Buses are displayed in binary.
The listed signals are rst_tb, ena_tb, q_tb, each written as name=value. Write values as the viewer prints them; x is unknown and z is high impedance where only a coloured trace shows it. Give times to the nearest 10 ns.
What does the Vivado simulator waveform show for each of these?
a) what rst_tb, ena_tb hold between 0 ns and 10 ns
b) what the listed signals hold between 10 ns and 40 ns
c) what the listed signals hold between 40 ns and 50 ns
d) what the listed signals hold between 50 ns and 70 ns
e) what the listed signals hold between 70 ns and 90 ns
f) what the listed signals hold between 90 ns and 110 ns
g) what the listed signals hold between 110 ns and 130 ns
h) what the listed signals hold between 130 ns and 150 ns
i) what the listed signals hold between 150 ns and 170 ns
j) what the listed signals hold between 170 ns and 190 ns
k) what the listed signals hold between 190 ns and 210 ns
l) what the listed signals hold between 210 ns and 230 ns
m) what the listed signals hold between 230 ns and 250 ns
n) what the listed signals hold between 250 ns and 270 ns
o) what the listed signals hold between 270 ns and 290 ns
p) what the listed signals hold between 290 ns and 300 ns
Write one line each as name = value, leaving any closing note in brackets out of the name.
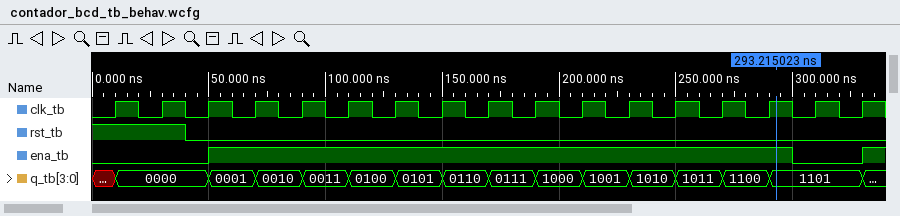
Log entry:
what rst_tb, ena_tb hold between 0 ns and 10 ns = rst_tb=1, ena_tb=0
what the listed signals hold between 10 ns and 40 ns = rst_tb=1, ena_tb=0, q_tb=0000
what the listed signals hold between 40 ns and 50 ns = rst_tb=0, ena_tb=0, q_tb=0000
what the listed signals hold between 50 ns and 70 ns = rst_tb=0, ena_tb=1, q_tb=0001
what the listed signals hold between 70 ns and 90 ns = rst_tb=0, ena_tb=1, q_tb=0010
what the listed signals hold between 90 ns and 110 ns = rst_tb=0, ena_tb=1, q_tb=0011
what the listed signals hold between 110 ns and 130 ns = rst_tb=0, ena_tb=1, q_tb=0100
what the listed signals hold between 130 ns and 150 ns = rst_tb=0, ena_tb=1, q_tb=0101
what the listed signals hold between 150 ns and 170 ns = rst_tb=0, ena_tb=1, q_tb=0110
what the listed signals hold between 170 ns and 190 ns = rst_tb=0, ena_tb=1, q_tb=0111
what the listed signals hold between 190 ns and 210 ns = rst_tb=0, ena_tb=1, q_tb=1000
what the listed signals hold between 210 ns and 230 ns = rst_tb=0, ena_tb=1, q_tb=1001
what the listed signals hold between 230 ns and 250 ns = rst_tb=0, ena_tb=1, q_tb=1010
what the listed signals hold between 250 ns and 270 ns = rst_tb=0, ena_tb=1, q_tb=1011
what the listed signals hold between 270 ns and 290 ns = rst_tb=0, ena_tb=1, q_tb=1100
what the listed signals hold between 290 ns and 300 ns = rst_tb=0, ena_tb=1, q_tb=1101
